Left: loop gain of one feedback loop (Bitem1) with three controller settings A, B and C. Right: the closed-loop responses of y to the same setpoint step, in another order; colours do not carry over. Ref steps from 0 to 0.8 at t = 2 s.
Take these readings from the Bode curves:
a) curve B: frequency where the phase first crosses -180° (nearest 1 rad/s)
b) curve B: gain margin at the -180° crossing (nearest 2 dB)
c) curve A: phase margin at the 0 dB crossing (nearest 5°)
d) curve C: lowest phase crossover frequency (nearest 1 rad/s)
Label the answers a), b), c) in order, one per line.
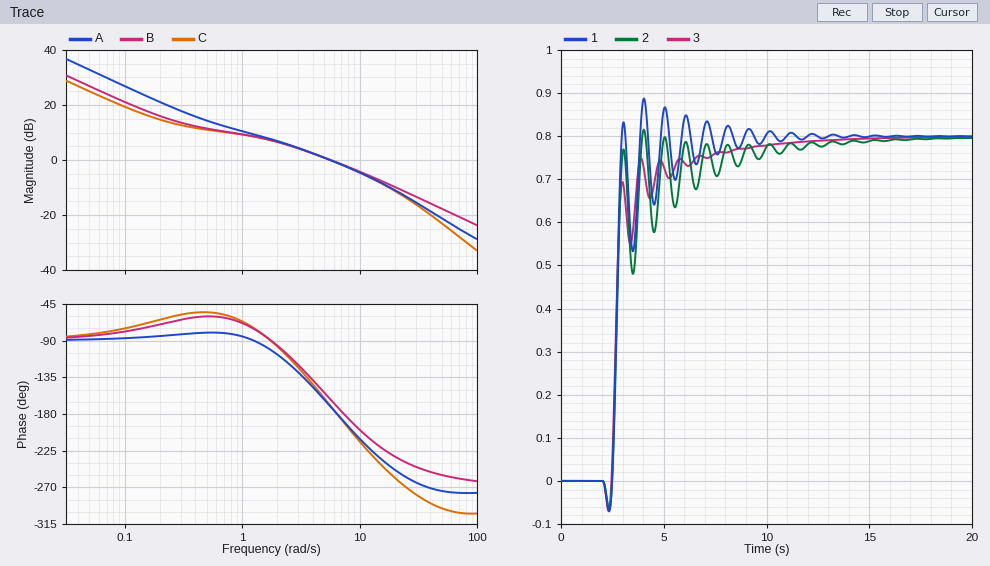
a) 7 rad/s
b) 2 dB
c) 10°
d) 6 rad/s
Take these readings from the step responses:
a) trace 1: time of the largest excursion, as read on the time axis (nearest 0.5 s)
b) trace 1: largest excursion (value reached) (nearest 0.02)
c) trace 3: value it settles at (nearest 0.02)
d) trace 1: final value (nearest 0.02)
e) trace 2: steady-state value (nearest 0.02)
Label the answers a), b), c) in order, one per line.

a) 4.0 s
b) 0.88
c) 0.80
d) 0.80
e) 0.80
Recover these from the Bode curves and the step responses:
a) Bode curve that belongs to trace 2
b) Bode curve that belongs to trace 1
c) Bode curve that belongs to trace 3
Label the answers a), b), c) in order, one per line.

a) C
b) A
c) B
